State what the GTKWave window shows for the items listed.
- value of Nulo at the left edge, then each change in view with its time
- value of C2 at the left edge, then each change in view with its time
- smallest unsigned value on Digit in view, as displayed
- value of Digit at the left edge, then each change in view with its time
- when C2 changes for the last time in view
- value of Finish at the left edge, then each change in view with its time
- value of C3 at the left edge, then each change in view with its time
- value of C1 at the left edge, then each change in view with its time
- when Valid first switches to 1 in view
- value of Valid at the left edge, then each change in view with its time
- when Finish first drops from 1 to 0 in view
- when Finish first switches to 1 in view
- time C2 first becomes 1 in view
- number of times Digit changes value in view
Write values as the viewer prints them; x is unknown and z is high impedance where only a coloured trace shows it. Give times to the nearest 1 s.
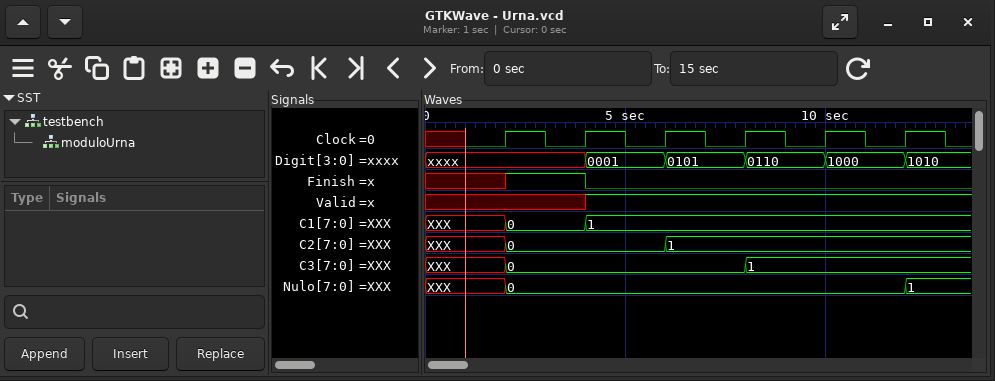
XXX, 0 at 2 s, 1 at 12 s
XXX, 0 at 2 s, 1 at 6 s
0001
xxxx, 0001 at 4 s, 0101 at 6 s, 0110 at 8 s, 1000 at 10 s, 1010 at 12 s
6 s
x, 1 at 2 s, 0 at 4 s
XXX, 0 at 2 s, 1 at 8 s
XXX, 0 at 2 s, 1 at 4 s
4 s
x, 1 at 4 s
4 s
2 s
6 s
5
